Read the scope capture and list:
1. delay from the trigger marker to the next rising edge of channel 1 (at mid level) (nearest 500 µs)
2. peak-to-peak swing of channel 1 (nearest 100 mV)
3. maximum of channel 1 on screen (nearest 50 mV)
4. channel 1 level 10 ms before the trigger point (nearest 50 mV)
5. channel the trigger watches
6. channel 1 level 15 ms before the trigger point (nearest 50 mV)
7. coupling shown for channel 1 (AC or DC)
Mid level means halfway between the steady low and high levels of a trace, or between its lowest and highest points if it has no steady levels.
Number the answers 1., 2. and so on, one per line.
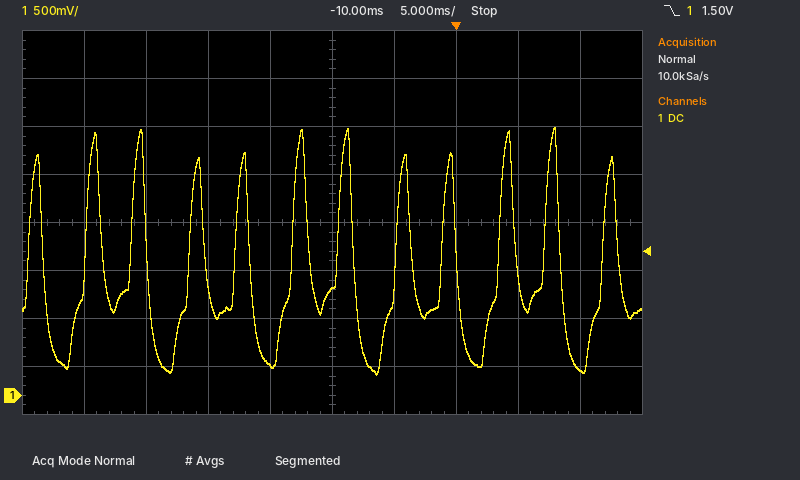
1. 3.5 ms
2. 2.60 V
3. 2.80 V
4. 1.10 V
5. channel 1
6. 300 mV
7. DC
